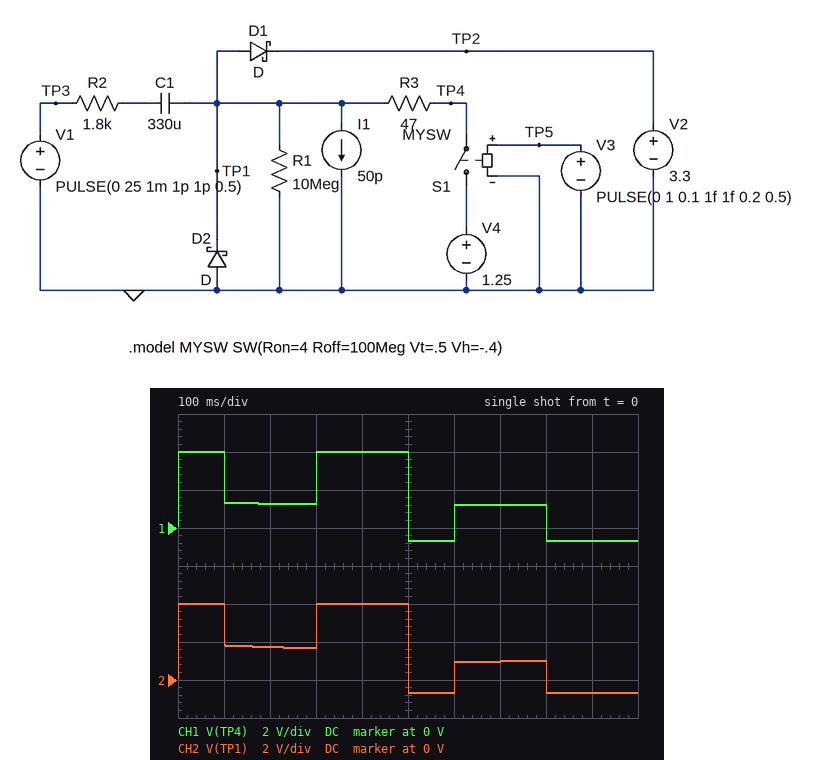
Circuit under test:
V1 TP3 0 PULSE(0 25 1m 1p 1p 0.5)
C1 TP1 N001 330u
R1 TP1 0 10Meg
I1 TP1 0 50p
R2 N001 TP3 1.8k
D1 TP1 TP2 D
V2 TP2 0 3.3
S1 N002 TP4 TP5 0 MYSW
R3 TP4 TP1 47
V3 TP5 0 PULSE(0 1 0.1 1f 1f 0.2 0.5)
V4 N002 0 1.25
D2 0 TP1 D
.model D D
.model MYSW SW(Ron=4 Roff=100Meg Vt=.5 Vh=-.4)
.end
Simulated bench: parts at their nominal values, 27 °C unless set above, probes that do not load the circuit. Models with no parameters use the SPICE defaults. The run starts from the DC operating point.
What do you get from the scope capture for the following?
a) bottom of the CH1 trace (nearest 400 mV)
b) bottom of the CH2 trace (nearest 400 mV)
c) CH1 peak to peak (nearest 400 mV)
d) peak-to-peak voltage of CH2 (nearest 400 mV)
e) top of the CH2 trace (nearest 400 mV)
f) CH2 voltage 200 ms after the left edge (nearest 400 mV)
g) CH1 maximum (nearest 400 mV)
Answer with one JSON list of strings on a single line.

["-800 mV", "-800 mV", "4.8 V", "4.8 V", "4.0 V", "1.6 V", "4.0 V"]
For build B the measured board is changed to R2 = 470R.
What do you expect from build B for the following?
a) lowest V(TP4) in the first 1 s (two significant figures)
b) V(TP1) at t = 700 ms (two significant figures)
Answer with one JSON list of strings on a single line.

["-750 mV", "570 mV"]
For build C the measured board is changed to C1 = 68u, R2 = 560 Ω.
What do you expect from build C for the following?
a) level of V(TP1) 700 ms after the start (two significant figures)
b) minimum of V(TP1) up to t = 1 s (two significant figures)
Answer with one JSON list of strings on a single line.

["1.2 V", "-750 mV"]
